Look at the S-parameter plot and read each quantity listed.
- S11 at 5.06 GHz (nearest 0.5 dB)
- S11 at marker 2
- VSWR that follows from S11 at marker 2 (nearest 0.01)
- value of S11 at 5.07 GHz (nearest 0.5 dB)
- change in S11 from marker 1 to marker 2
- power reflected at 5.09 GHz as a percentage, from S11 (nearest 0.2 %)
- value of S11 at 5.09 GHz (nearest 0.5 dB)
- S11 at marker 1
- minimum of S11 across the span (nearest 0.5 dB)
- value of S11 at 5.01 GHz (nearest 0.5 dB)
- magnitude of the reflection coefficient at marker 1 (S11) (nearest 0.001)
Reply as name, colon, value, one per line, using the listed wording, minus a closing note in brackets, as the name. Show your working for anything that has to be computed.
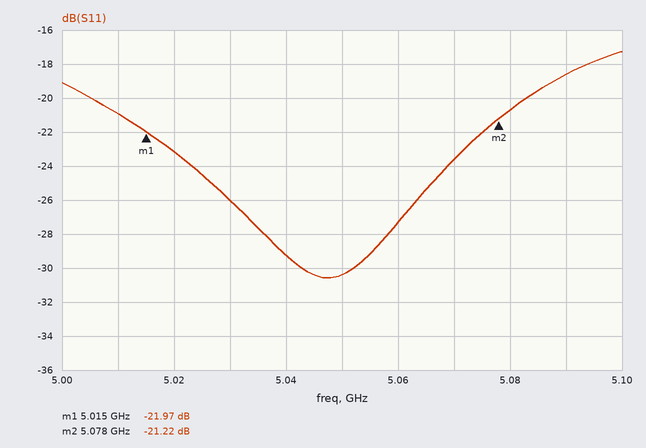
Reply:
S11 at 5.06 GHz: -27.5 dB
S11 at marker 2: -21.22 dB
VSWR that follows from S11 at marker 2: (1 + 0.0869)/(1 − 0.0869) ≈ 1.19
value of S11 at 5.07 GHz: -23.5 dB
change in S11 from marker 1 to marker 2: -21.22 − (-21.97) = 0.75 dB
power reflected at 5.09 GHz as a percentage, from S11: 10^(-18.5/10) ≈ 1.4 %
value of S11 at 5.09 GHz: -18.5 dB
S11 at marker 1: -21.97 dB
minimum of S11 across the span: -30.5 dB
value of S11 at 5.01 GHz: -21.0 dB
magnitude of the reflection coefficient at marker 1 (S11): 10^(-21.97/20) ≈ 0.080
